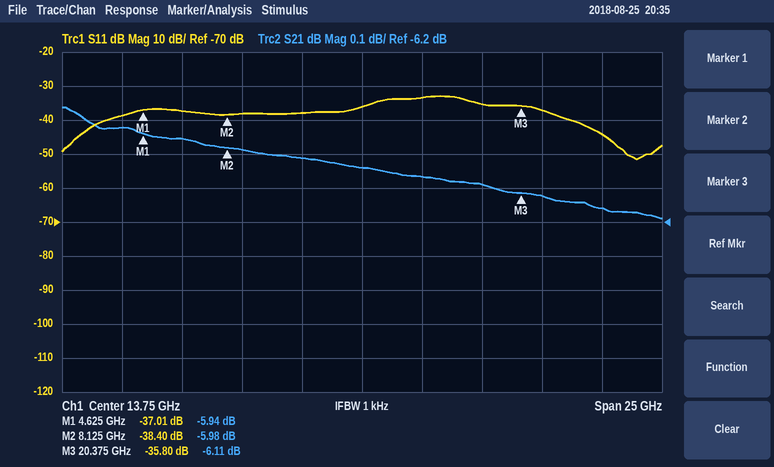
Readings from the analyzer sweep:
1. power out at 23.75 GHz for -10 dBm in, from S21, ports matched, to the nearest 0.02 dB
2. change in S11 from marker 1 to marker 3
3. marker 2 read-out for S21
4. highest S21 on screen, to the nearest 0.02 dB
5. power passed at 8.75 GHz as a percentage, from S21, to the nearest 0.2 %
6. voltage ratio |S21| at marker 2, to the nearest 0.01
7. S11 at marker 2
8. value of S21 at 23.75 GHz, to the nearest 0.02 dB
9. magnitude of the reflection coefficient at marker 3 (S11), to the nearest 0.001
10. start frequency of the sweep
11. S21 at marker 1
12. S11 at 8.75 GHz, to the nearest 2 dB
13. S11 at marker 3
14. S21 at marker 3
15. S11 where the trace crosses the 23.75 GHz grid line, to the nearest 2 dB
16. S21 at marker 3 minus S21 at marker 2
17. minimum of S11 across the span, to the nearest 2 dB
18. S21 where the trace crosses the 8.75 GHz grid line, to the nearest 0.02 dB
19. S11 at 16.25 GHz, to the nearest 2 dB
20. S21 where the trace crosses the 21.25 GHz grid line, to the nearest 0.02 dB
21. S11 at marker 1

-16.16 dBm
1.21 dB
-5.98 dB
-5.86 dB
25.2 %
0.50
-38.40 dB
-6.16 dB
0.016
1.25 GHz
-5.94 dB
-38 dB
-35.80 dB
-6.11 dB
-44 dB
-0.13 dB
-52 dB
-5.98 dB
-34 dB
-6.12 dB
-37.01 dB
